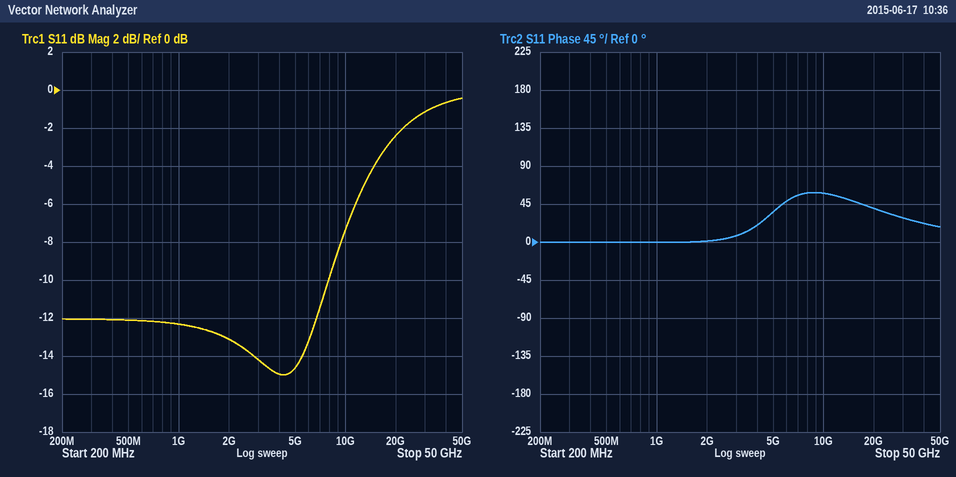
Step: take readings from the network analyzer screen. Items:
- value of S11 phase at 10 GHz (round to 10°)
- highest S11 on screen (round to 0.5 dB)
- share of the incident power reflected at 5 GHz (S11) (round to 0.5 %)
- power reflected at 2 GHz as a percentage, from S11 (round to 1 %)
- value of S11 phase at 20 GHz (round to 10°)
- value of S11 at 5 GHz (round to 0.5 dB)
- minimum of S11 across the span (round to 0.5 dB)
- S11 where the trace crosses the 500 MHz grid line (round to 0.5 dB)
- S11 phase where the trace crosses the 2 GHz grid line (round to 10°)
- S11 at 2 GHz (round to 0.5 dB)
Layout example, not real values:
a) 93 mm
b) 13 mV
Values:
a) 60°
b) -0.5 dB
c) 3.5 %
d) 5 %
e) 40°
f) -14.5 dB
g) -15.0 dB
h) -12.0 dB
i) 0°
j) -13.0 dB
